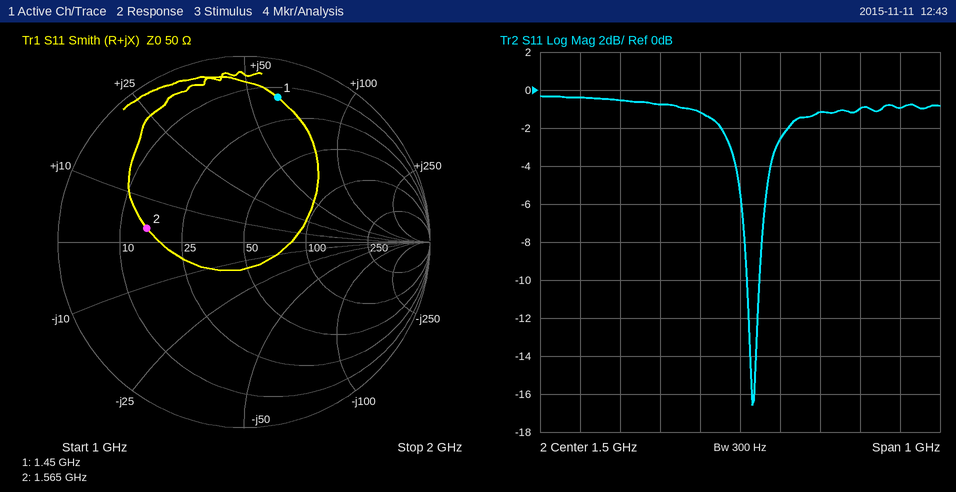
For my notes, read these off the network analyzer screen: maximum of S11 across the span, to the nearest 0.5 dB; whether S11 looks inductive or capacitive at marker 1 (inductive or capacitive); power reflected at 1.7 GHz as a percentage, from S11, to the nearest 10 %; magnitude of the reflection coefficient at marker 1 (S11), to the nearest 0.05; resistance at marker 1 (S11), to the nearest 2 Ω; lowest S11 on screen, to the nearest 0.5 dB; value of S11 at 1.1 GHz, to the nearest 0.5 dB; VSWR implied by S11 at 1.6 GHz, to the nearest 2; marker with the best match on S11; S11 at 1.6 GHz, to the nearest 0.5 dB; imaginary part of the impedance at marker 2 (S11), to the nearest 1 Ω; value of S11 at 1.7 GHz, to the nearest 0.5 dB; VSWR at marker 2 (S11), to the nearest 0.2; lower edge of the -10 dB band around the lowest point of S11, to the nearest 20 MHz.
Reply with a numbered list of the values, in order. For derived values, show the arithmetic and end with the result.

1. -0.5 dB
2. inductive
3. 10^(-1/10) ≈ 79.4 %, so 80 % to the nearest 10 %
4. 0.80
5. 14 Ω
6. -16.5 dB
7. -0.5 dB
8. |Γ| = 10^(-2.5/20) = 0.7499; VSWR = (1 + 0.7499)/(1 − 0.7499) ≈ 7.00, so 6 to the nearest 2
9. marker 2
10. -2.5 dB
11. +3 Ω
12. -1.0 dB
13. 3.2
14. 1.52 GHz
